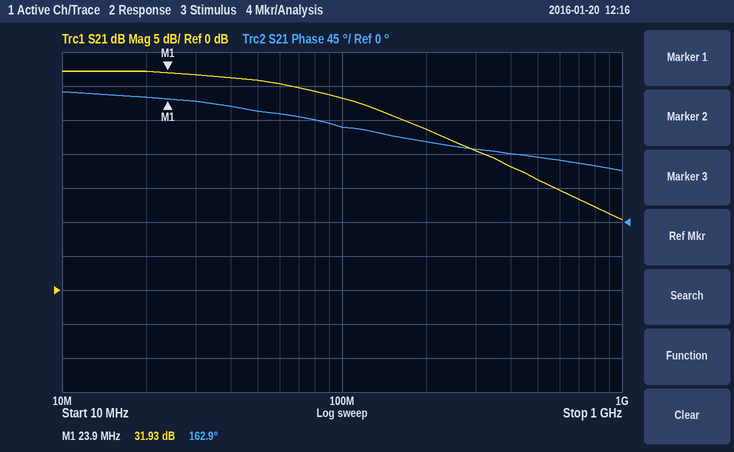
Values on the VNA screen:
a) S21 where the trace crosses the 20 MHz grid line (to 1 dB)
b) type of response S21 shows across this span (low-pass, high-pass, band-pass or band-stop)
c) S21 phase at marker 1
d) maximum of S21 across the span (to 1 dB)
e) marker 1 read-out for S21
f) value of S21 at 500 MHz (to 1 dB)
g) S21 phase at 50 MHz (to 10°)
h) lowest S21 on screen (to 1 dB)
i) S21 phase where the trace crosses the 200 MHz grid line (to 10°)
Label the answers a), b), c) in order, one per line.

a) 32 dB
b) low-pass
c) 162.9°
d) 32 dB
e) 31.93 dB
f) 16 dB
g) 150°
h) 10 dB
i) 110°
